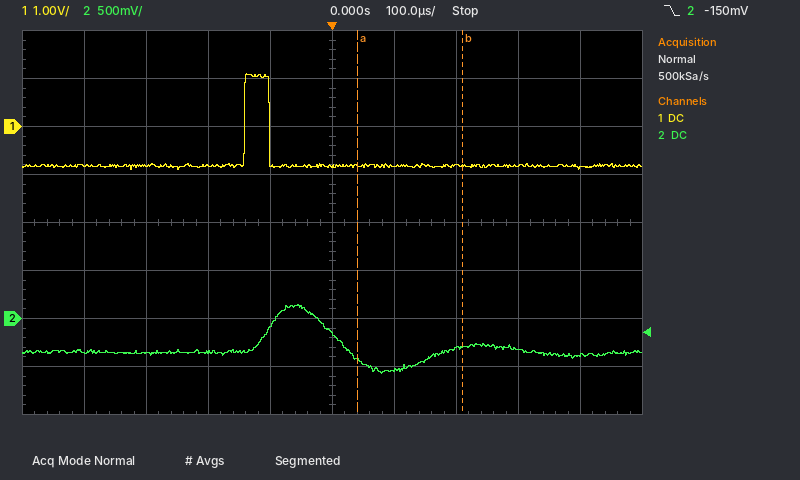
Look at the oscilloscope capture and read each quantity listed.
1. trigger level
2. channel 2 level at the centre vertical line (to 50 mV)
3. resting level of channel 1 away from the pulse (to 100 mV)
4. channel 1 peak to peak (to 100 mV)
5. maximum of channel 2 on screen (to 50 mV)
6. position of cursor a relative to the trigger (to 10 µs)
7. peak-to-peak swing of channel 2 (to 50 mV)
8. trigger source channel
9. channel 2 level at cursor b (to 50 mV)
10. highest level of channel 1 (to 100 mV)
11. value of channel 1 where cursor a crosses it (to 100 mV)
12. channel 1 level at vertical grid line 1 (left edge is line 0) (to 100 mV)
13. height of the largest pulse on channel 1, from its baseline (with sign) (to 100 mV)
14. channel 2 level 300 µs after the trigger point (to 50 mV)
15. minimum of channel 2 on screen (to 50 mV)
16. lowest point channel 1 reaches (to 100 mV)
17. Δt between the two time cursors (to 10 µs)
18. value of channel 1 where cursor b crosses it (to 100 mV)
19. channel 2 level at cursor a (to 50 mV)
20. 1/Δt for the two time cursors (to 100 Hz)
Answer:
-150 mV
-150 mV
-800 mV
2.0 V
150 mV
+40 µs
700 mV
channel 2
-300 mV
1.1 V
-800 mV
-800 mV
+1.9 V
-300 mV
-550 mV
-900 mV
170 µs
-800 mV
-450 mV
5.9 kHz
